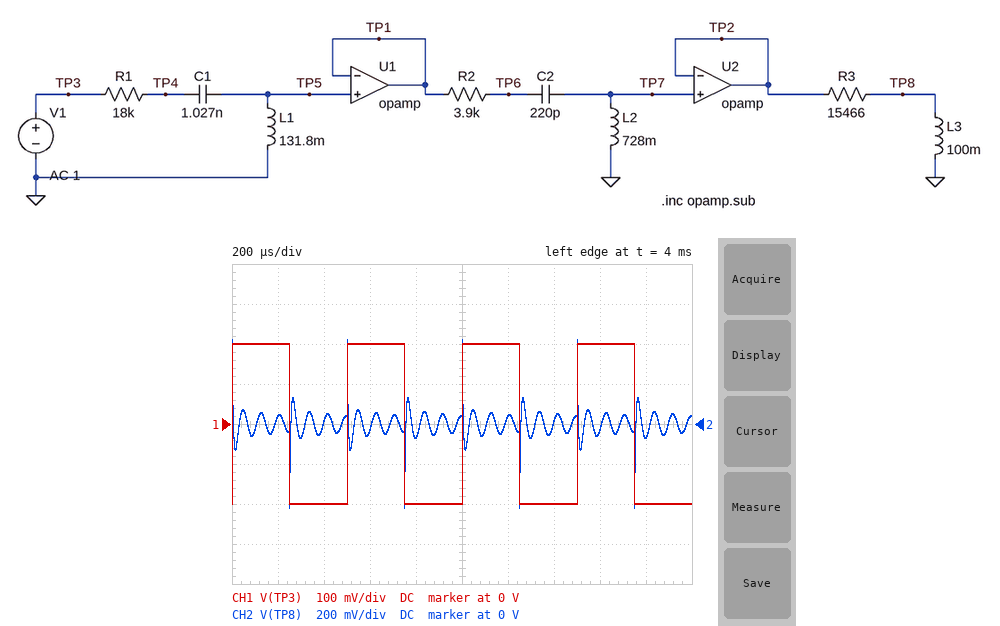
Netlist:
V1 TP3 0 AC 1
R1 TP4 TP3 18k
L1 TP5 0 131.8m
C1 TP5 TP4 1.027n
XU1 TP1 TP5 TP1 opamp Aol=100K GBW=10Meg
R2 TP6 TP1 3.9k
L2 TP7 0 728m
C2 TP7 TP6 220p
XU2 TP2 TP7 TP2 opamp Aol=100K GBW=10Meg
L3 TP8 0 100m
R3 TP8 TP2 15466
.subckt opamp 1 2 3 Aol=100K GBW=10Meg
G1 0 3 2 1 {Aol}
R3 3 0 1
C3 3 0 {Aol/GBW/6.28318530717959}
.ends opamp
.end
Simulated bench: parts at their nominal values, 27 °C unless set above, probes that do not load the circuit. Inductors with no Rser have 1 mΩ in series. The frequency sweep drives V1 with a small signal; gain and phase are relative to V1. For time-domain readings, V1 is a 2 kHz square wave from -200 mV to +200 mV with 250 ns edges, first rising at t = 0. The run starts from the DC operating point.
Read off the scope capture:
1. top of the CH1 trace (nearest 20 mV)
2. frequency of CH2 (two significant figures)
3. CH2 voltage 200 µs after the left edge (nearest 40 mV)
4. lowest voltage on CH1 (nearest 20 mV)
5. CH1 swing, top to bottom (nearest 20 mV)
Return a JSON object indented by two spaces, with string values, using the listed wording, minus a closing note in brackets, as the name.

{
  "top of the CH1 trace": "200 mV",
  "frequency of CH2": "2.0 kHz",
  "CH2 voltage 200 µs after the left edge": "40 mV",
  "lowest voltage on CH1": "-200 mV",
  "CH1 swing, top to bottom": "400 mV"
}
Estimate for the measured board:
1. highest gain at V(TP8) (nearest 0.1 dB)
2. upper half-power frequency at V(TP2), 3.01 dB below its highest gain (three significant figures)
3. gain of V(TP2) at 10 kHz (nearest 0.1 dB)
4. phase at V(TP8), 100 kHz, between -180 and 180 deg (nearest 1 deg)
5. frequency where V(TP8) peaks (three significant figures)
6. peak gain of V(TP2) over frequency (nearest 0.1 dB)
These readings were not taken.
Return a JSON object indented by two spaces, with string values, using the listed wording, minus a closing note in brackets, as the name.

{
  "highest gain at V(TP8)": "11.8 dB",
  "upper half-power frequency at V(TP2), 3.01 dB below its highest gain": "13.1 kHz",
  "gain of V(TP2) at 10 kHz": "-2.8 dB",
  "phase at V(TP8), 100 kHz, between -180 and 180 deg": "26 deg",
  "frequency where V(TP8) peaks": "12.6 kHz",
  "peak gain of V(TP2) over frequency": "18.6 dB"
}
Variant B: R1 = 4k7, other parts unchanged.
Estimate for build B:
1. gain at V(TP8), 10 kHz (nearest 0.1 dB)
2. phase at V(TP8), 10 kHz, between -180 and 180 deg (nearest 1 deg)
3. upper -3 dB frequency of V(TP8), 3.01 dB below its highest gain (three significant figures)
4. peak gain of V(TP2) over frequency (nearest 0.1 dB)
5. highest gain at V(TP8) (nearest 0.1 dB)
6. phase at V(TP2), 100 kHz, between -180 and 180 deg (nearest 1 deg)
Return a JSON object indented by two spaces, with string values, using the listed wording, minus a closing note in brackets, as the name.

{
  "gain at V(TP8), 10 kHz": "-4.2 dB",
  "phase at V(TP8), 10 kHz, between -180 and 180 deg": "26 deg",
  "upper -3 dB frequency of V(TP8), 3.01 dB below its highest gain": "13.2 kHz",
  "peak gain of V(TP2) over frequency": "29.7 dB",
  "highest gain at V(TP8)": "22.9 dB",
  "phase at V(TP2), 100 kHz, between -180 and 180 deg": "3 deg"
}
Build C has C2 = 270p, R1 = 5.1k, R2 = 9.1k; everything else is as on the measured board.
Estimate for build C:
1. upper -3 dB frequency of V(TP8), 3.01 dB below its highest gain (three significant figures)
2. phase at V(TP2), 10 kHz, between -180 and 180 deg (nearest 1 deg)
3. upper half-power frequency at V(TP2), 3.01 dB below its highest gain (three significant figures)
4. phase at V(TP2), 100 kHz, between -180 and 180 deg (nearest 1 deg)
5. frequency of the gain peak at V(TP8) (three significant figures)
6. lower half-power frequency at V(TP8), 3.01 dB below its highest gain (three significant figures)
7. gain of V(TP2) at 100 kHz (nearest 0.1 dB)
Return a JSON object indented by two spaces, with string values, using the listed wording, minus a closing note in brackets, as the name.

{
  "upper -3 dB frequency of V(TP8), 3.01 dB below its highest gain": "14.9 kHz",
  "phase at V(TP2), 10 kHz, between -180 and 180 deg": "-70 deg",
  "upper half-power frequency at V(TP2), 3.01 dB below its highest gain": "14.0 kHz",
  "phase at V(TP2), 100 kHz, between -180 and 180 deg": "4 deg",
  "frequency of the gain peak at V(TP8)": "11.9 kHz",
  "lower half-power frequency at V(TP8), 3.01 dB below its highest gain": "11.0 kHz",
  "gain of V(TP2) at 100 kHz": "0.3 dB"
}
